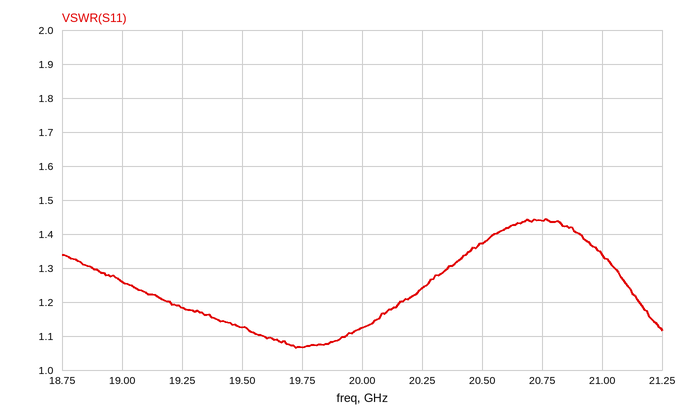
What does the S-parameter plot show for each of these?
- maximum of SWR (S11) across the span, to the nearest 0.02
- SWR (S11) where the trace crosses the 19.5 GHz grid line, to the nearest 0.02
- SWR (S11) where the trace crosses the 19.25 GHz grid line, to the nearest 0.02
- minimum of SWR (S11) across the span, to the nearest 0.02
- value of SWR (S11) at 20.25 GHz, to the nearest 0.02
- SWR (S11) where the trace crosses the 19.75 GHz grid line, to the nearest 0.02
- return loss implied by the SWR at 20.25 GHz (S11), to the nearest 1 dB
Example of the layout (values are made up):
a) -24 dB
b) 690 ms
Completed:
a) 1.44
b) 1.12
c) 1.18
d) 1.06
e) 1.24
f) 1.06
g) 19 dB
